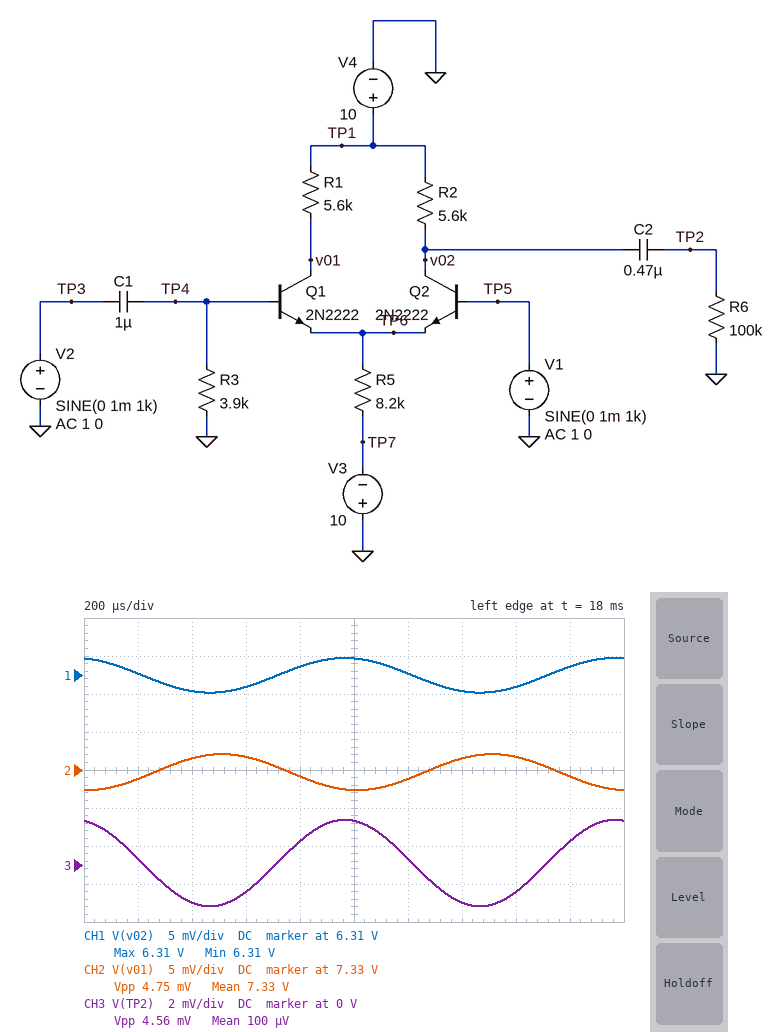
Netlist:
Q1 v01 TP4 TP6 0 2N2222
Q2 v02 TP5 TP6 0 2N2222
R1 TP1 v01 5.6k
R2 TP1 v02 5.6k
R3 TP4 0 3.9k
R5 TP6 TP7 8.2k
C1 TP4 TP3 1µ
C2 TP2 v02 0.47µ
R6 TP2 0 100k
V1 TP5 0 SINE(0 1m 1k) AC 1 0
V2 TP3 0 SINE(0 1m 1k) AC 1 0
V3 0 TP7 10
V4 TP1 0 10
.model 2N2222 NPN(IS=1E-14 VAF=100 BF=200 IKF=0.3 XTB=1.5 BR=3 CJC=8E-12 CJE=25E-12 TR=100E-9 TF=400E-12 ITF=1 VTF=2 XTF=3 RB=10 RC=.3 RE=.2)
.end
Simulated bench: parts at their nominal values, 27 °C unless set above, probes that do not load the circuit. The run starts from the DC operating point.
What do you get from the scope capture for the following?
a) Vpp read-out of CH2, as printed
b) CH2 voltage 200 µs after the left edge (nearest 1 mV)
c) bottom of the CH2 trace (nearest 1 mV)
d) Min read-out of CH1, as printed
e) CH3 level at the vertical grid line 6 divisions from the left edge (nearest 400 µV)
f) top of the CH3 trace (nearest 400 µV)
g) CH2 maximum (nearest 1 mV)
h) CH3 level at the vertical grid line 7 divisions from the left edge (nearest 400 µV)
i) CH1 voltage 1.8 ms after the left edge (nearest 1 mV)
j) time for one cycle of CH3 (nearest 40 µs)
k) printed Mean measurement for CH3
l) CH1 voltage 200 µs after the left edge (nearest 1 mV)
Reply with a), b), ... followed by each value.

a) 4.75 mV
b) 7.329 V
c) 7.327 V
d) 6.31 V
e) 400 µV
f) 2.4 mV
g) 7.332 V
h) -2.0 mV
i) 6.311 V
j) 1.00 ms
k) 100 µV
l) 6.310 V
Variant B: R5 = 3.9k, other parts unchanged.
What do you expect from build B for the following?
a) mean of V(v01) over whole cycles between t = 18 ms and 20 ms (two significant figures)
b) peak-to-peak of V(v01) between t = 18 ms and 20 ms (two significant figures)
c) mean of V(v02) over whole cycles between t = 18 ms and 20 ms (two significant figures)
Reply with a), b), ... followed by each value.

a) 5.2 V
b) 9.1 mV
c) 1.5 V
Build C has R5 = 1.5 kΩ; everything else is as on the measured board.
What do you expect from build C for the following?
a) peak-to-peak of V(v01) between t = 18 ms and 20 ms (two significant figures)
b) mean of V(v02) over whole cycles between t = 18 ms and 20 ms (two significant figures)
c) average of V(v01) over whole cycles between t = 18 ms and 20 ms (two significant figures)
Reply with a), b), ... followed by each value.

a) 3.0 mV
b) -730 mV
c) -630 mV
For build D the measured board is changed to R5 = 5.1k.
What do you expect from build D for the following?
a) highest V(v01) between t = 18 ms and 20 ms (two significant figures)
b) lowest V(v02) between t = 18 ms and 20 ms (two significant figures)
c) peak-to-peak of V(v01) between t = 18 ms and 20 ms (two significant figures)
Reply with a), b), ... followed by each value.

a) 6.1 V
b) 3.7 V
c) 7.2 mV
